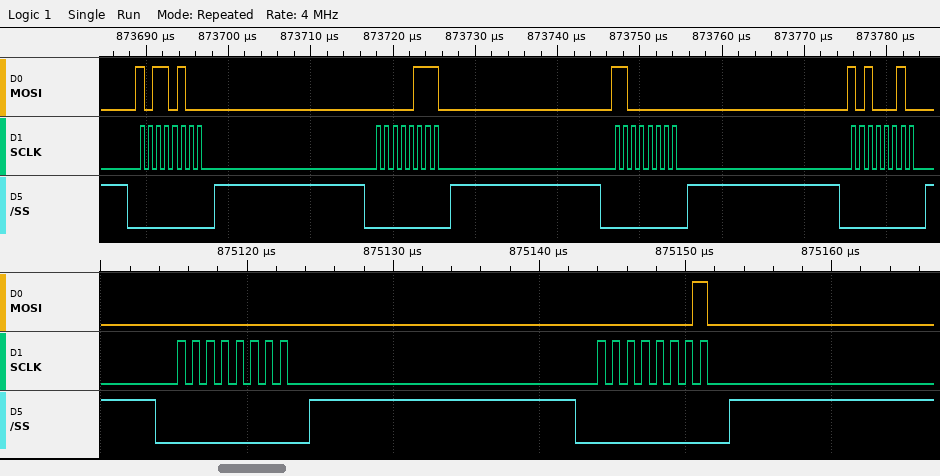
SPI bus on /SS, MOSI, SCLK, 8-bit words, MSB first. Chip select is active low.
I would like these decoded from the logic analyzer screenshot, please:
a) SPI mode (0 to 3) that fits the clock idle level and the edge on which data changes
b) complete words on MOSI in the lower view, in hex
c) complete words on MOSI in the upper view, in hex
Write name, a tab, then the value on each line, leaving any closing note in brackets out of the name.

SPI mode (0 to 3) that fits the clock idle level and the edge on which data changes	0
complete words on MOSI in the lower view, in hex	00, 01
complete words on MOSI in the upper view, in hex	B4, 07, C0, A2
